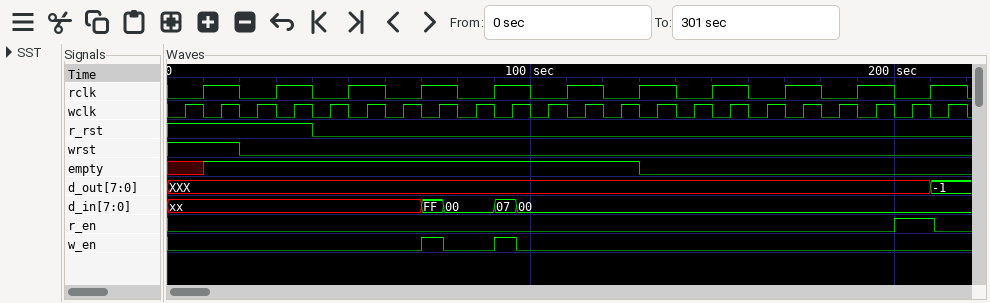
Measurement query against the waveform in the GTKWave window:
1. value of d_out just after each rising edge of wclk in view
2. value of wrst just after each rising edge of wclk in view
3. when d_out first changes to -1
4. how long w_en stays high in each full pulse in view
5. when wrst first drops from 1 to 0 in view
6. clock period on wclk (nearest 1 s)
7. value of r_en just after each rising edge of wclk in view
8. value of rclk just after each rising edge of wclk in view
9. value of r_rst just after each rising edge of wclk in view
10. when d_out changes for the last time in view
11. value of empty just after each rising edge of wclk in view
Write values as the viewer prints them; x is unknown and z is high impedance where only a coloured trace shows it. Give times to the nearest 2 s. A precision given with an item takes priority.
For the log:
XXX, XXX, XXX, XXX, XXX, XXX, XXX, XXX, XXX, XXX, XXX, XXX, XXX, XXX, XXX, XXX, XXX, XXX, XXX, XXX, XXX, -1
1 1 0 0 0 0 0 0 0 0 0 0 0 0 0 0 0 0 0 0 0 0
210 s
6 s, 6 s
20 s
10 s
0 0 0 0 0 0 0 0 0 0 0 0 0 0 0 0 0 0 0 0 1 0
0 1 0 1 0 1 0 1 0 1 0 1 0 1 0 1 0 1 0 1 0 1
1 1 1 1 0 0 0 0 0 0 0 0 0 0 0 0 0 0 0 0 0 0
210 s
x 1 1 1 1 1 1 1 1 1 1 1 1 0 0 0 0 0 0 0 0 0
